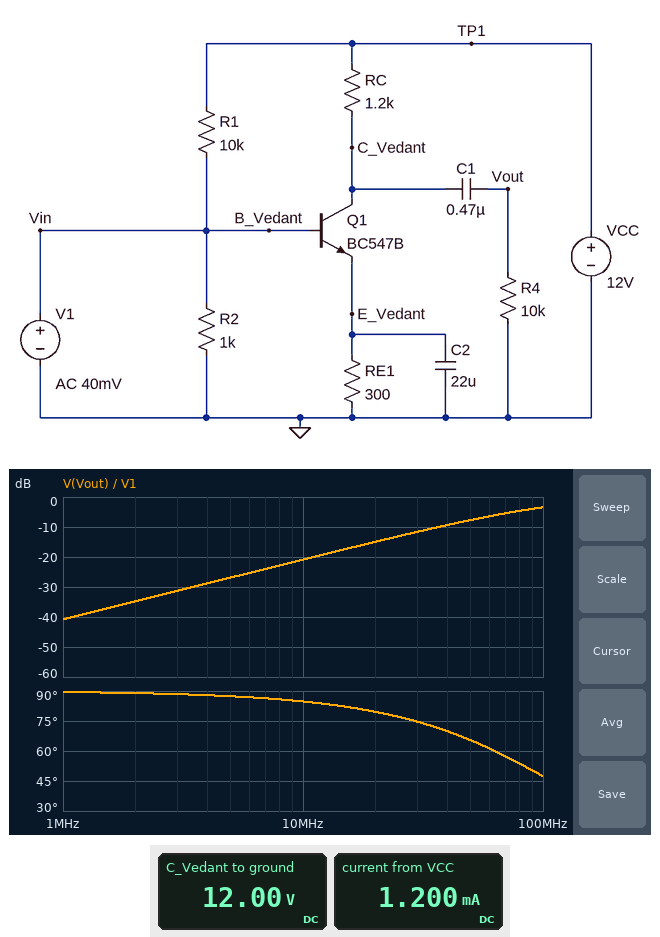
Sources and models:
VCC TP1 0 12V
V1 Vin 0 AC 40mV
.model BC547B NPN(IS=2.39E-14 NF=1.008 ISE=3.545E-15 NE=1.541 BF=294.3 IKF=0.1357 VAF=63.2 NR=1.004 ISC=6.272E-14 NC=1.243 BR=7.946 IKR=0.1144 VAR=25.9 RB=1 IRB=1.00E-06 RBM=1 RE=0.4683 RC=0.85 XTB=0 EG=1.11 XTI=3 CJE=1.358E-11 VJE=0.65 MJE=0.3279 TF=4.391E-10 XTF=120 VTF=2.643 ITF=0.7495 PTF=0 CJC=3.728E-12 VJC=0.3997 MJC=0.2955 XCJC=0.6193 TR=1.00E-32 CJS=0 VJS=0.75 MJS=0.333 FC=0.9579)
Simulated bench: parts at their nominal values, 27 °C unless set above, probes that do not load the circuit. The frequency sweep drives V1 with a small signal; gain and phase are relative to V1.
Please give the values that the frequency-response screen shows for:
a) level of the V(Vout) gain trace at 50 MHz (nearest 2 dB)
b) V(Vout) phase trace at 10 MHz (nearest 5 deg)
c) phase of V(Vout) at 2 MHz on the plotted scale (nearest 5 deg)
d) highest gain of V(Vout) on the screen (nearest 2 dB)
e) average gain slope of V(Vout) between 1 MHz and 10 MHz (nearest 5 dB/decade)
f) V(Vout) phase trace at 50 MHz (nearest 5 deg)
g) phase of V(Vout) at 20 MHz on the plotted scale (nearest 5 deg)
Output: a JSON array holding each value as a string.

["-8 dB", "85 deg", "90 deg", "-4 dB", "20 dB/decade", "65 deg", "80 deg"]
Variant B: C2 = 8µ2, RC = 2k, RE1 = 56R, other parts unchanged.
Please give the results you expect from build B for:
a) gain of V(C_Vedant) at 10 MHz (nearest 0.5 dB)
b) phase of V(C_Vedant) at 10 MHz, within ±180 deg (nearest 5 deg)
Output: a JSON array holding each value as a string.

["-17.0 dB", "80 deg"]
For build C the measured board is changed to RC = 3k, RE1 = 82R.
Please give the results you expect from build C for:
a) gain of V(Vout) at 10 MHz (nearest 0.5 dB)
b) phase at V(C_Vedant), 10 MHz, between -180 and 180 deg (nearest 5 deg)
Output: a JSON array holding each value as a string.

["-14.5 dB", "80 deg"]
